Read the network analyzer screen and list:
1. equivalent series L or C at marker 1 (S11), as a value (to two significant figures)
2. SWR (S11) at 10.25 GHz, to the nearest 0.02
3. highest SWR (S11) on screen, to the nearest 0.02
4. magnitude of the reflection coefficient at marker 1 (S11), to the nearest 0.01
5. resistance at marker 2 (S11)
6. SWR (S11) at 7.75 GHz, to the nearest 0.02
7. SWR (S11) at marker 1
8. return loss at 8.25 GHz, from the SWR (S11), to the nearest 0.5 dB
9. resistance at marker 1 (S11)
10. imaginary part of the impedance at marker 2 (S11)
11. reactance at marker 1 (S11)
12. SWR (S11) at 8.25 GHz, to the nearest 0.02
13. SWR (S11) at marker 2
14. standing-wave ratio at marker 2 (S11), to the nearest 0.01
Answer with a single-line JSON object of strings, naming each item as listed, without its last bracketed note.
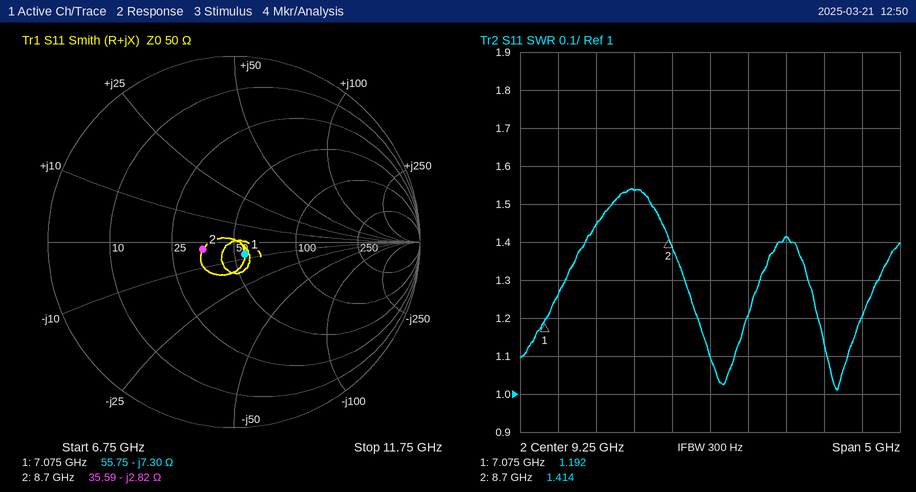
{"equivalent series L or C at marker 1 (S11), as a value": "3.1 pF", "SWR (S11) at 10.25 GHz, to the nearest 0.02": "1.42", "highest SWR (S11) on screen, to the nearest 0.02": "1.54", "magnitude of the reflection coefficient at marker 1 (S11), to the nearest 0.01": "0.09", "resistance at marker 2": "35.59 Ω", "SWR (S11) at 7.75 GHz, to the nearest 0.02": "1.44", "SWR (S11) at marker 1": "1.192", "return loss at 8.25 GHz, from the SWR (S11), to the nearest 0.5 dB": "13.5 dB", "resistance at marker 1": "55.75 Ω", "imaginary part of the impedance at marker 2": "-2.82 Ω", "reactance at marker 1": "-7.30 Ω", "SWR (S11) at 8.25 GHz, to the nearest 0.02": "1.54", "SWR (S11) at marker 2": "1.414", "standing-wave ratio at marker 2 (S11), to the nearest 0.01": "1.41"}
